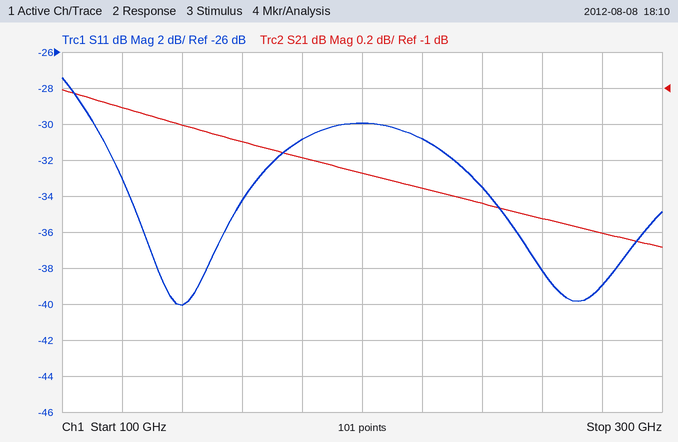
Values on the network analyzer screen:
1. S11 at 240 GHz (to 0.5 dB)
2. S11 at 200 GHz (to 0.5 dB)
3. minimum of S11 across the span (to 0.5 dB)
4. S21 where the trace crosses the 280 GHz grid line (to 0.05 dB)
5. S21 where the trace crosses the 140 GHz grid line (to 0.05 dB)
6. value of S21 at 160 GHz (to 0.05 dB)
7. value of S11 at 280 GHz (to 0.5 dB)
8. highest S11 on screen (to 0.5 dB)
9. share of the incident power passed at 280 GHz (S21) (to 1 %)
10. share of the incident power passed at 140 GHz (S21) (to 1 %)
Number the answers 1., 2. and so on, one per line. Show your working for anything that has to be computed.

1. -33.5 dB
2. -30.0 dB
3. -40.0 dB
4. -1.80 dB
5. -1.20 dB
6. -1.30 dB
7. -39.0 dB
8. -27.5 dB
9. 10^(-1.8/10) ≈ 66 %
10. 10^(-1.2/10) ≈ 76 %
